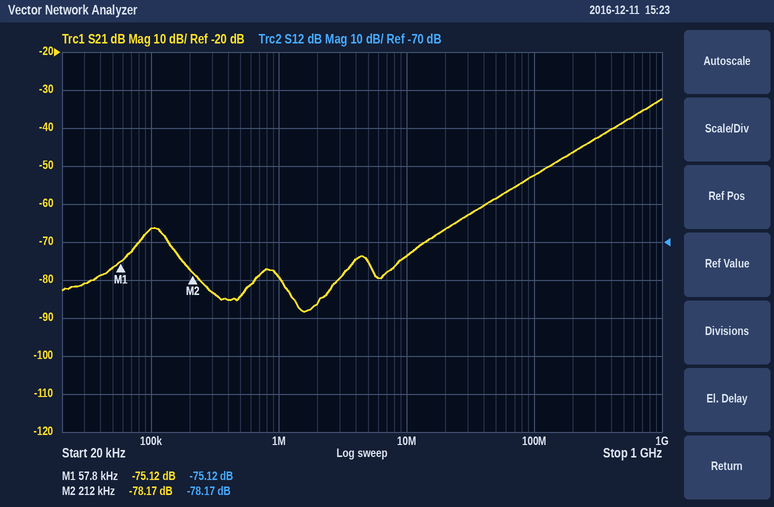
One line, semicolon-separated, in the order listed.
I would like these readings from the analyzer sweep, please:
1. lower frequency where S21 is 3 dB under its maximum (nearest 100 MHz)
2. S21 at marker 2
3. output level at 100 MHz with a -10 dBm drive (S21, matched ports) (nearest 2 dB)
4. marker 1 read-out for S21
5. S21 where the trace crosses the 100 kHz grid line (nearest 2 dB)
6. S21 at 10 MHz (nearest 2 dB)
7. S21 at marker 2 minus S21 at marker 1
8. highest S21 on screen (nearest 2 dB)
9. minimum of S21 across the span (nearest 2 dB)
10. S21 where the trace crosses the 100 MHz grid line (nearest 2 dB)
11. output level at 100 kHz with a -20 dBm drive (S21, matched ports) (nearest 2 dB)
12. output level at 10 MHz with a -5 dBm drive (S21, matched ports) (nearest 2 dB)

700 MHz; -78.17 dB; -62 dBm; -75.12 dB; -66 dB; -74 dB; -3.05 dB; -32 dB; -88 dB; -52 dB; -86 dBm; -78 dBm
